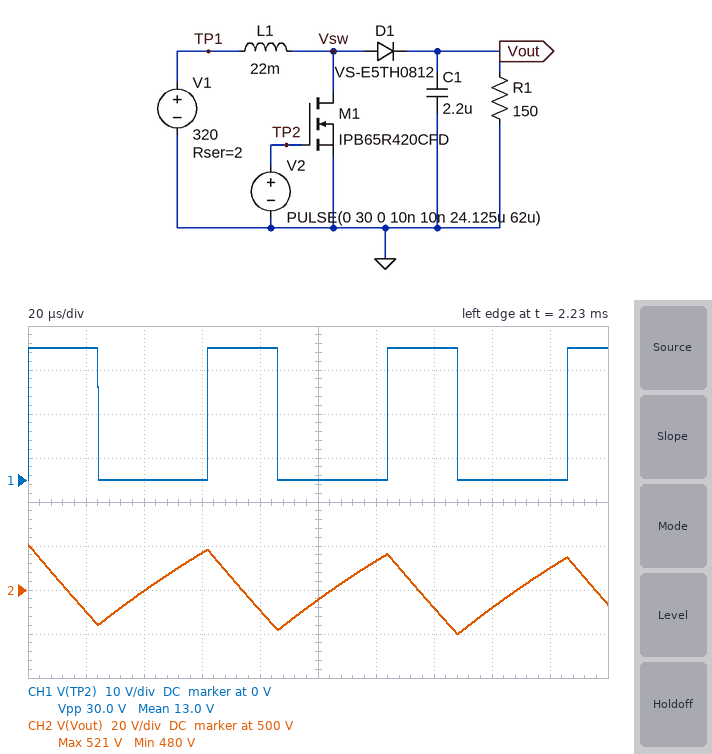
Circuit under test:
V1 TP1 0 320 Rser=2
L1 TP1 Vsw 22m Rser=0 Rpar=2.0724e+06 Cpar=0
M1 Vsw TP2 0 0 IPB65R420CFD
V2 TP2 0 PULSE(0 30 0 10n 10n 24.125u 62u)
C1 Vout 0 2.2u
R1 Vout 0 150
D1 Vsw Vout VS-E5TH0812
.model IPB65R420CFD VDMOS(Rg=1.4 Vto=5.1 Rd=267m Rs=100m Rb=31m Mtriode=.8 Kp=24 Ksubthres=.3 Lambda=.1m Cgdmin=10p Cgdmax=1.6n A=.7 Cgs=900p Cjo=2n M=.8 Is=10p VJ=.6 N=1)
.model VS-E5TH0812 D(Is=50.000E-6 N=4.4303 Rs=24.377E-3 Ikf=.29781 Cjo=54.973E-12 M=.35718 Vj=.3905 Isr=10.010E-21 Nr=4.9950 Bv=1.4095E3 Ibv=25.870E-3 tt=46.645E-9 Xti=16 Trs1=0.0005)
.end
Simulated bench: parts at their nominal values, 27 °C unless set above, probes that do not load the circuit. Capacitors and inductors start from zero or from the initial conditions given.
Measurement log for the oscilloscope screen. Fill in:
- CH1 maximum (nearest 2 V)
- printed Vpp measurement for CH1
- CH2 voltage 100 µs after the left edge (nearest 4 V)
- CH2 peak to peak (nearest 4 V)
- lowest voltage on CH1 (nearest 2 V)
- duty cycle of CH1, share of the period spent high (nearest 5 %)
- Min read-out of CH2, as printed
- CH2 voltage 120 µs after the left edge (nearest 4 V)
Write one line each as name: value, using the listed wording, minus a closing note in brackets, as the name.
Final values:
CH1 maximum: 30 V
printed Vpp measurement for CH1: 30.0 V
CH2 voltage 100 µs after the left edge: 496 V
CH2 peak to peak: 40 V
lowest voltage on CH1: 0 V
duty cycle of CH1, share of the period spent high: 40 %
Min read-out of CH2, as printed: 480 V
CH2 voltage 120 µs after the left edge: 512 V
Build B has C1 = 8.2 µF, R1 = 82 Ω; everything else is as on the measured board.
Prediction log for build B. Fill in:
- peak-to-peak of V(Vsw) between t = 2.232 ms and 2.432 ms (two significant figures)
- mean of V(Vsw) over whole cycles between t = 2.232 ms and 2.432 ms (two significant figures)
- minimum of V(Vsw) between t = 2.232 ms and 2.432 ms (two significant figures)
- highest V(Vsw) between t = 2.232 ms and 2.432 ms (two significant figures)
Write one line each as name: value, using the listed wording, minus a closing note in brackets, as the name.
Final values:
peak-to-peak of V(Vsw) between t = 2.232 ms and 2.432 ms: 560 V
mean of V(Vsw) over whole cycles between t = 2.232 ms and 2.432 ms: 340 V
minimum of V(Vsw) between t = 2.232 ms and 2.432 ms: 3.6 V
highest V(Vsw) between t = 2.232 ms and 2.432 ms: 570 V
